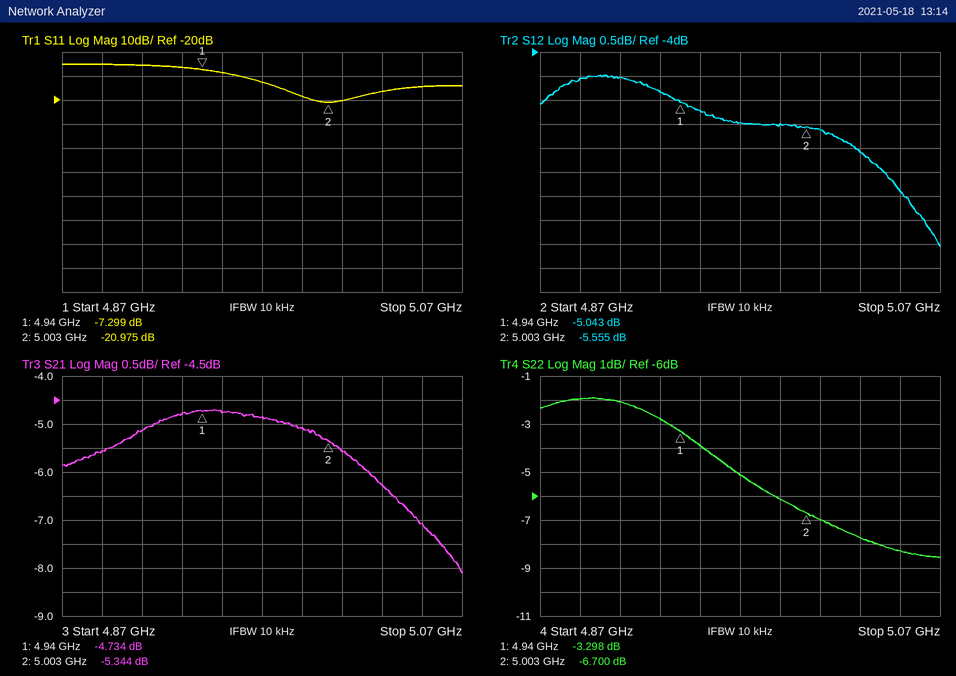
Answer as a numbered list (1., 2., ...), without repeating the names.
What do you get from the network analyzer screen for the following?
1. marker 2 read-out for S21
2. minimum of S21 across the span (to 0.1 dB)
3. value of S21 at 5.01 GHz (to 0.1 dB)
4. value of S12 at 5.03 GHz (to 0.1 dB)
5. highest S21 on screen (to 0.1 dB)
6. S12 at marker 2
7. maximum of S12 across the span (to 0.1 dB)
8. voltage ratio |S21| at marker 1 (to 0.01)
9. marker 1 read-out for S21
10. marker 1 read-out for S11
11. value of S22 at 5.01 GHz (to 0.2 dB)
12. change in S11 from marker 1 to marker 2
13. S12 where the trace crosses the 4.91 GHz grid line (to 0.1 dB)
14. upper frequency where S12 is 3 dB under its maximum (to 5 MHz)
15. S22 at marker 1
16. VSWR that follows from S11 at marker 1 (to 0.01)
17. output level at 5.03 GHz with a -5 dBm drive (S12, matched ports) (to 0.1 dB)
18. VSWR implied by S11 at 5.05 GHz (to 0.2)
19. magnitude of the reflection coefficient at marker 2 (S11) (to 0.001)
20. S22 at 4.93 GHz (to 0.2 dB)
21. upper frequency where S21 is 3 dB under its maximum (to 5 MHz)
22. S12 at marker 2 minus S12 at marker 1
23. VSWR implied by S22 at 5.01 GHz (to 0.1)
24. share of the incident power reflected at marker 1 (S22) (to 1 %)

1. -5.344 dB
2. -8.1 dB
3. -5.6 dB
4. -6.1 dB
5. -4.7 dB
6. -5.555 dB
7. -4.5 dB
8. 0.58
9. -4.734 dB
10. -7.299 dB
11. -7.0 dB
12. -13.676 dB
13. -4.5 dB
14. 5.060 GHz
15. -3.298 dB
16. 2.52
17. -11.1 dBm
18. 1.4
19. 0.089
20. -2.8 dB
21. 5.065 GHz
22. -0.512 dB
23. 2.6
24. 47 %
